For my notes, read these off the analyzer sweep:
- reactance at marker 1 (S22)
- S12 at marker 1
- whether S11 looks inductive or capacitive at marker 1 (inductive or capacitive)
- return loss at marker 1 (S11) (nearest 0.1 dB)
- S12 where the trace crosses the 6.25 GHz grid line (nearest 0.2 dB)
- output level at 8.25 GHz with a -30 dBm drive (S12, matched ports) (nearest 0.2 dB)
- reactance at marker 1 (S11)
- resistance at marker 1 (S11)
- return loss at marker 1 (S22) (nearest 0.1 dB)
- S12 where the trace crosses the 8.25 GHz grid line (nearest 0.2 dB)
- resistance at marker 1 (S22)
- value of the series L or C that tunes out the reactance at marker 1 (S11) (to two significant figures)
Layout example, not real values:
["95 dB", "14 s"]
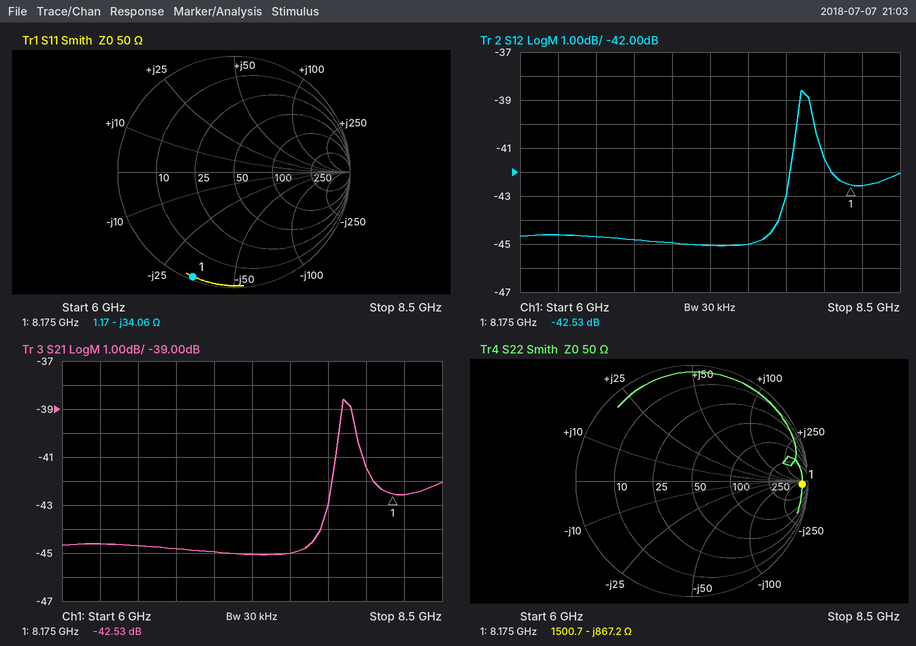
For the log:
["-867.2 Ω", "-42.53 dB", "capacitive", "0.3 dB", "-44.6 dB", "-72.6 dBm", "-34.06 Ω", "1.17 Ω", "0.4 dB", "-42.6 dB", "1500.7 Ω", "660 pH"]
